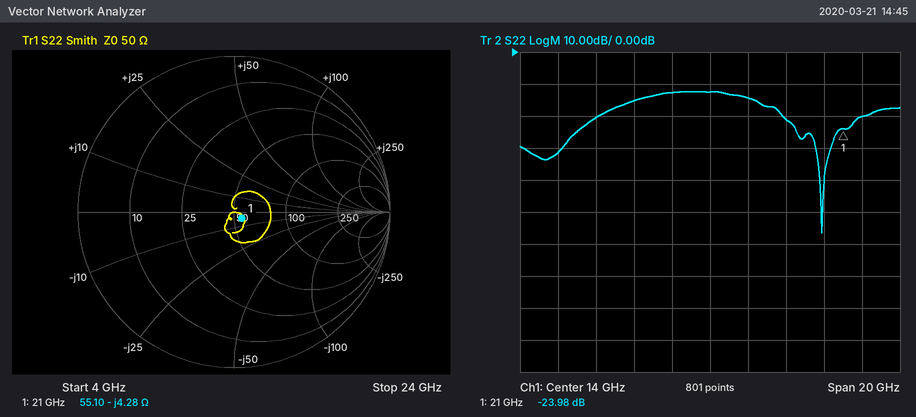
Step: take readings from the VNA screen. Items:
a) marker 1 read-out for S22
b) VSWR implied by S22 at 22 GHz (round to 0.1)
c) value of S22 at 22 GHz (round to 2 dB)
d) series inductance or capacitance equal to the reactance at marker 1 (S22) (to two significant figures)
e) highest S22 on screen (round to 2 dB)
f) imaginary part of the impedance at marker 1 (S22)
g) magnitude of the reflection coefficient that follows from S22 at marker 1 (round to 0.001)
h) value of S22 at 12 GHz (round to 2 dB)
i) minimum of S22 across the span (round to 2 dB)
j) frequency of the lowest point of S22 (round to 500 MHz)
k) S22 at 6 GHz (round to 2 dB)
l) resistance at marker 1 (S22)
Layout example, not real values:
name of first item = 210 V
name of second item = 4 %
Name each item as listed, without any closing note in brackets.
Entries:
marker 1 read-out for S22 = -23.98 dB
VSWR implied by S22 at 22 GHz = 1.2
value of S22 at 22 GHz = -20 dB
series inductance or capacitance equal to the reactance at marker 1 (S22) = 1.8 pF
highest S22 on screen = -12 dB
imaginary part of the impedance at marker 1 = -4.28 Ω
magnitude of the reflection coefficient that follows from S22 at marker 1 = 0.063
value of S22 at 12 GHz = -12 dB
minimum of S22 across the span = -56 dB
frequency of the lowest point of S22 = 20.0 GHz
S22 at 6 GHz = -32 dB
resistance at marker 1 = 55.10 Ω
